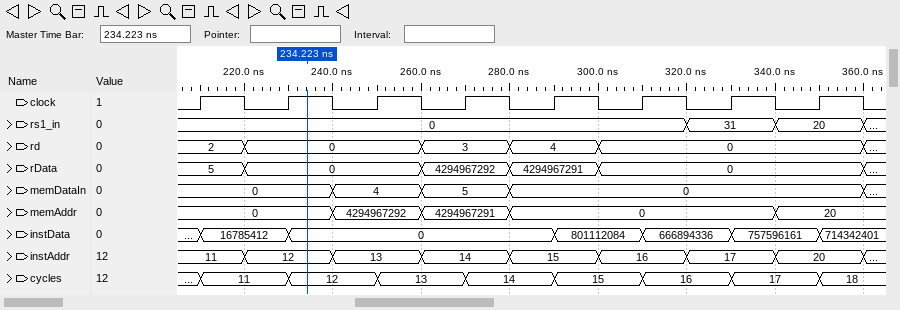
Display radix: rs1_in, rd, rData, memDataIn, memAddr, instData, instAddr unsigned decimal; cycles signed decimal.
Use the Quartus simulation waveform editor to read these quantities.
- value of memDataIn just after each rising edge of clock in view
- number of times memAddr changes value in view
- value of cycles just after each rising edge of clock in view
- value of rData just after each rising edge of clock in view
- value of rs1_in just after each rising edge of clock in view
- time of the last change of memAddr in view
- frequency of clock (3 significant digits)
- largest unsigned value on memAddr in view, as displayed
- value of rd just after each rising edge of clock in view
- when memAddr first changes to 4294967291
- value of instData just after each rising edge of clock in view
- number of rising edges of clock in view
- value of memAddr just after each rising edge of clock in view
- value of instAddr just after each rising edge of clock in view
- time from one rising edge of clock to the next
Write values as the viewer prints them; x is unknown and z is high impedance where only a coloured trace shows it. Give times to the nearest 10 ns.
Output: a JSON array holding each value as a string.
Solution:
["0, 0, 4, 5, 0, 0, 0, 0", "4", "11, 12, 13, 14, 15, 16, 17, 18", "5, 0, 0, 4294967292, 4294967291, 0, 0, 0", "0, 0, 0, 0, 0, 0, 31, 20", "340 ns", "50.0 MHz", "4294967292", "2, 0, 0, 3, 4, 0, 0, 0", "260 ns", "16785412, 0, 0, 0, 801112084, 666894336, 757596161, 714342401", "8", "0, 0, 4294967292, 4294967291, 0, 0, 0, 20", "11, 12, 13, 14, 15, 16, 17, 20", "20 ns"]
